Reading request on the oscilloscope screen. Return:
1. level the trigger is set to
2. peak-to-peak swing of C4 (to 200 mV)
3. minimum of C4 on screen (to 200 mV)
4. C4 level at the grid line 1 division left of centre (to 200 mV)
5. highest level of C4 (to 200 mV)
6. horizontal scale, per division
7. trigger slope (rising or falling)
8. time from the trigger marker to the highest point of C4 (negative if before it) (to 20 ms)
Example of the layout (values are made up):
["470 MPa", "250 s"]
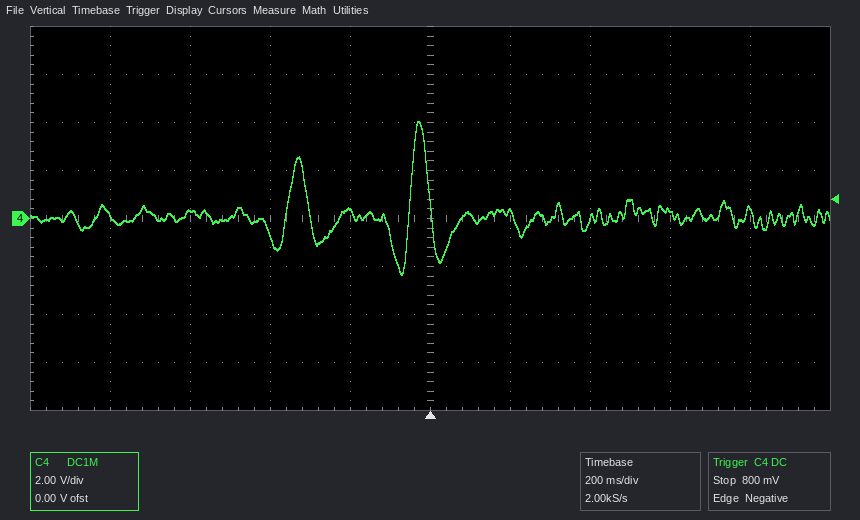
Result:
["800 mV", "6.4 V", "-2.4 V", "200 mV", "4.0 V", "200 ms", "falling", "-20 ms"]
